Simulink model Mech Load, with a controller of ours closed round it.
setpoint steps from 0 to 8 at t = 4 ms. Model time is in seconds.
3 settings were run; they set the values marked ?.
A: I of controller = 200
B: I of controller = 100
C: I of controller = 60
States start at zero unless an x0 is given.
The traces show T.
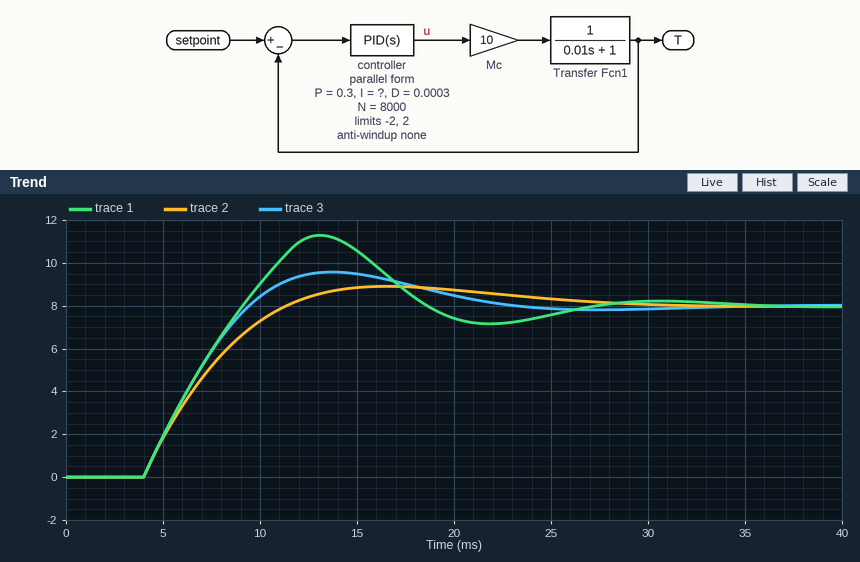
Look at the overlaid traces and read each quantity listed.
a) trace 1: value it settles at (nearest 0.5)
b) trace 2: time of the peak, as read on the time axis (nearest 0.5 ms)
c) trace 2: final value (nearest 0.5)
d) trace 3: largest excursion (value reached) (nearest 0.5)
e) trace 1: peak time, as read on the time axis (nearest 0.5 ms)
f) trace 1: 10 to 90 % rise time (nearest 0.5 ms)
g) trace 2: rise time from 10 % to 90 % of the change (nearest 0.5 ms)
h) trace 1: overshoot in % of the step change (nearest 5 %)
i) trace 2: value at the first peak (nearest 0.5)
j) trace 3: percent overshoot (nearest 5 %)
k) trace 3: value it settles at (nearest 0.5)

8.0
16.5 ms
8.0
9.5
13.0 ms
4.0 ms
5.5 ms
40 %
9.0
20 %
8.0
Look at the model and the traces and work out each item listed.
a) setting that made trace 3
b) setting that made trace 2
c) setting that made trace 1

B
C
A
